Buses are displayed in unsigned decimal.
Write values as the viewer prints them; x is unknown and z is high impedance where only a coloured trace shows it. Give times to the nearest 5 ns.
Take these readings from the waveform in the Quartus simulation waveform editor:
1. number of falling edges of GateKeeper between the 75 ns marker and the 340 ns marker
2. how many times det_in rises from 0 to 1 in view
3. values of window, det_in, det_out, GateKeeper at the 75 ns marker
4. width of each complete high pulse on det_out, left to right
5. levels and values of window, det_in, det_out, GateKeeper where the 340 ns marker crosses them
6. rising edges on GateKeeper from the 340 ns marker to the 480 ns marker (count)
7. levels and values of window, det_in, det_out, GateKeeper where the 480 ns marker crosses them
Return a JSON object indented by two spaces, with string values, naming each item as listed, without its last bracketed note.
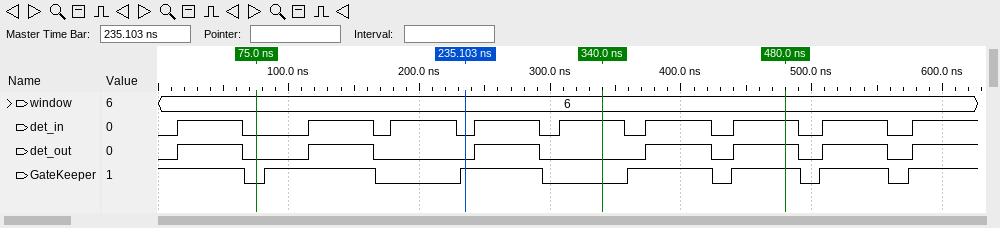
{
  "number of falling edges of GateKeeper between the 75 ns marker and the 340 ns marker": "2",
  "how many times det_in rises from 0 to 1 in view": "9",
  "values of window, det_in, det_out, GateKeeper at the 75 ns marker": "window=6, det_in=0, det_out=0, GateKeeper=0",
  "width of each complete high pulse on det_out, left to right": "50 ns, 50 ns, 50 ns, 50 ns, 50 ns, 50 ns",
  "levels and values of window, det_in, det_out, GateKeeper where the 340 ns marker crosses them": "window=6, det_in=1, det_out=0, GateKeeper=0",
  "rising edges on GateKeeper from the 340 ns marker to the 480 ns marker": "2",
  "levels and values of window, det_in, det_out, GateKeeper where the 480 ns marker crosses them": "window=6, det_in=1, det_out=1, GateKeeper=1"
}
